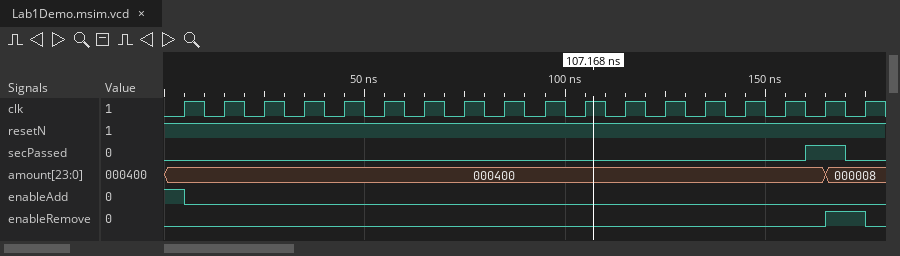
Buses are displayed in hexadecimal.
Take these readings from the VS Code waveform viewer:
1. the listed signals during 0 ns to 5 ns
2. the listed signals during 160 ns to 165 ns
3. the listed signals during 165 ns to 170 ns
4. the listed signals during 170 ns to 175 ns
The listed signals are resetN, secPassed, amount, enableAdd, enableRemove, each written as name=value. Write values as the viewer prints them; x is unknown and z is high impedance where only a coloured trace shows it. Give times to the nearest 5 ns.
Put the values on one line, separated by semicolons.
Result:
resetN=1, secPassed=0, amount=000400, enableAdd=1, enableRemove=0; resetN=1, secPassed=1, amount=000400, enableAdd=0, enableRemove=0; resetN=1, secPassed=1, amount=000008, enableAdd=0, enableRemove=1; resetN=1, secPassed=0, amount=000008, enableAdd=0, enableRemove=1
